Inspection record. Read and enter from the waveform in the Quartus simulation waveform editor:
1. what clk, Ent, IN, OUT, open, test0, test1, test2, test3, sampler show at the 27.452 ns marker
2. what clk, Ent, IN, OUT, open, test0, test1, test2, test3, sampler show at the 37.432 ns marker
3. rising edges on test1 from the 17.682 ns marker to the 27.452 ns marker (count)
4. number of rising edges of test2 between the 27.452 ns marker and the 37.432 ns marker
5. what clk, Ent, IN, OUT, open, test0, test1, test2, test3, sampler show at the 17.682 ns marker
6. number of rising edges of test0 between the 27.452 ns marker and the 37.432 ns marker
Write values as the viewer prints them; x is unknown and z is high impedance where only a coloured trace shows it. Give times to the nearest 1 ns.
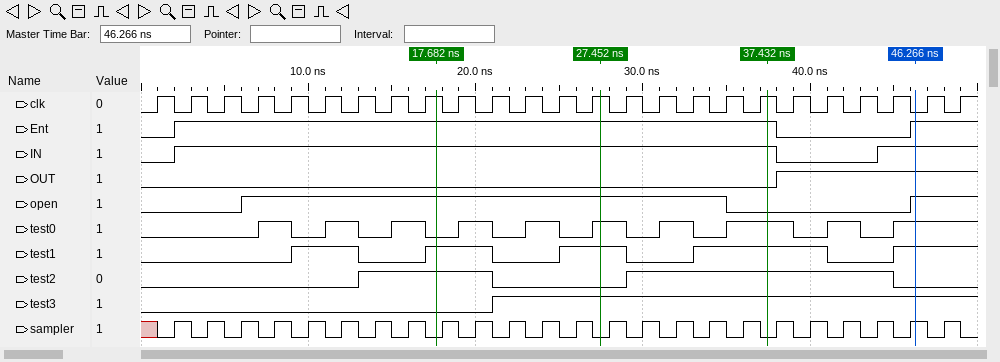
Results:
clk=1, Ent=1, IN=1, OUT=0, open=1, test0=1, test1=1, test2=0, test3=1, sampler=0
clk=1, Ent=1, IN=1, OUT=0, open=0, test0=1, test1=1, test2=1, test3=1, sampler=0
1
1
clk=1, Ent=1, IN=1, OUT=0, open=1, test0=0, test1=1, test2=1, test3=0, sampler=0
2
